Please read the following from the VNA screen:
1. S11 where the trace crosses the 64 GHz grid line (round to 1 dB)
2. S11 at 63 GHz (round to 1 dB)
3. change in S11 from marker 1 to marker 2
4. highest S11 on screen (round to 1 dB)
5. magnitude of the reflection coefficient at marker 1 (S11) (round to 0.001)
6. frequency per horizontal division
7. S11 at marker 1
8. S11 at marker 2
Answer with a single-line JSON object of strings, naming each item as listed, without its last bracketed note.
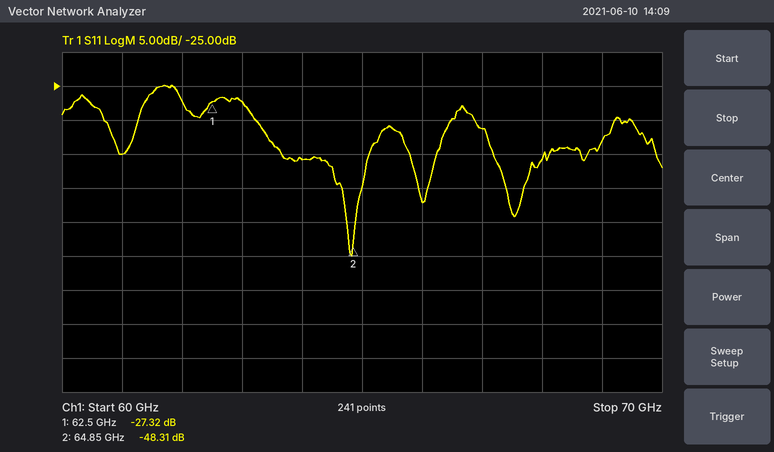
{"S11 where the trace crosses the 64 GHz grid line": "-36 dB", "S11 at 63 GHz": "-27 dB", "change in S11 from marker 1 to marker 2": "-20.99 dB", "highest S11 on screen": "-25 dB", "magnitude of the reflection coefficient at marker 1 (S11)": "0.043", "frequency per horizontal division": "1 GHz", "S11 at marker 1": "-27.32 dB", "S11 at marker 2": "-48.31 dB"}
